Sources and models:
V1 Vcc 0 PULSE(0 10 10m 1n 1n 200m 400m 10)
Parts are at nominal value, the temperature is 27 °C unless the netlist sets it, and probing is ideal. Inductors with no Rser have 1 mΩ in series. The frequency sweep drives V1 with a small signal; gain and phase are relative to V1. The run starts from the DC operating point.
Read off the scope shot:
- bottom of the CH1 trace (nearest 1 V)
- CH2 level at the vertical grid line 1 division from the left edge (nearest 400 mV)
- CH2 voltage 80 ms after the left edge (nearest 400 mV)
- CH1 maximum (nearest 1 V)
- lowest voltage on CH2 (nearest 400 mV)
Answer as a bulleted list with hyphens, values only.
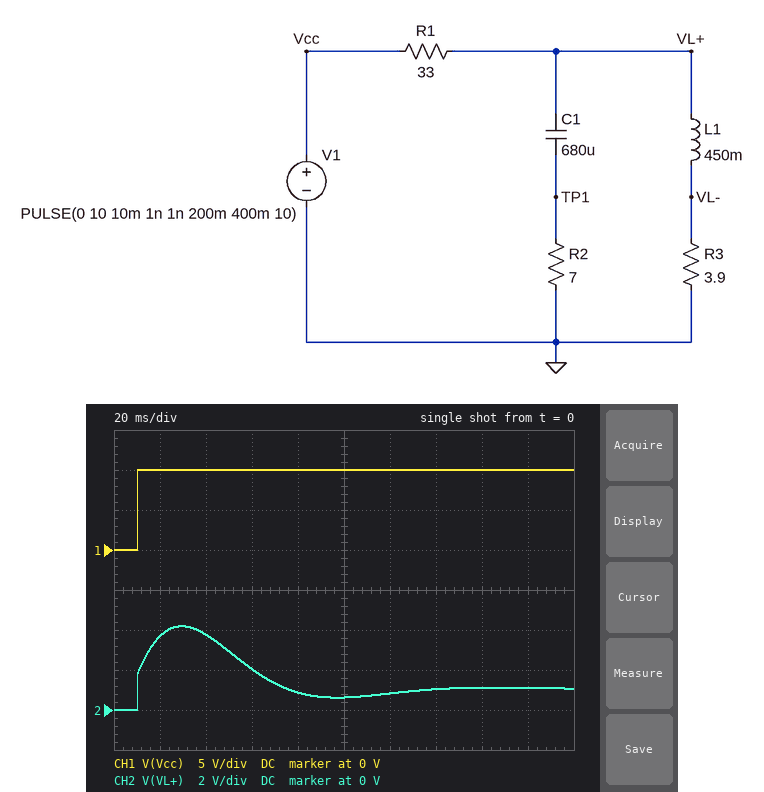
- 0 V
- 3.6 V
- 800 mV
- 10 V
- 0 V
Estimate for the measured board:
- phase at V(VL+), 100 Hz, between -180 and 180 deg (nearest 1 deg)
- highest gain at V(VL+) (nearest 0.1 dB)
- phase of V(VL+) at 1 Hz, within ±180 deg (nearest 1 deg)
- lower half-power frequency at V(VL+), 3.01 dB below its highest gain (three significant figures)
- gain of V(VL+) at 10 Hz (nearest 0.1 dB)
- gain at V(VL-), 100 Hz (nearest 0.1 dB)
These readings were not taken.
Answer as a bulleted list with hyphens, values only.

- -14 deg
- -3.6 dB
- 31 deg
- 5.26 Hz
- -3.8 dB
- -51.9 dB
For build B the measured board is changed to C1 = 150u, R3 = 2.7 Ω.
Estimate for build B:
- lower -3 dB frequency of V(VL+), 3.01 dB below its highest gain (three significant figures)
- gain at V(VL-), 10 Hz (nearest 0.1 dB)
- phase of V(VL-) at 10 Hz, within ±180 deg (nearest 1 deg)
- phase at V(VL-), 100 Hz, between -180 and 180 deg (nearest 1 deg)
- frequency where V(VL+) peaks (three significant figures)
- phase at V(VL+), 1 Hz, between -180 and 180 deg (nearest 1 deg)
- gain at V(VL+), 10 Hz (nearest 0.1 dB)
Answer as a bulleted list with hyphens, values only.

- 8.76 Hz
- -23.4 dB
- -48 deg
- -130 deg
- 18.4 Hz
- 42 deg
- -3.0 dB
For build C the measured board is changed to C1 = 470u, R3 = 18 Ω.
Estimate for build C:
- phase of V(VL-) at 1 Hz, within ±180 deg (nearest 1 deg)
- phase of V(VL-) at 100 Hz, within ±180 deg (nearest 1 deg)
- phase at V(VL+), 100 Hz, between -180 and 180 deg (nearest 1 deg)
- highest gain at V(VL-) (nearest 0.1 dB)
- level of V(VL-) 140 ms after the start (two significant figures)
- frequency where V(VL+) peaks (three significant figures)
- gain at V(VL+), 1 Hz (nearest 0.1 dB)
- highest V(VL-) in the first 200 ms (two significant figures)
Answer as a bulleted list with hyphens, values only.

- -5 deg
- -106 deg
- -20 deg
- -9.0 dB
- 3.5 V
- 11.3 Hz
- -8.9 dB
- 3.7 V
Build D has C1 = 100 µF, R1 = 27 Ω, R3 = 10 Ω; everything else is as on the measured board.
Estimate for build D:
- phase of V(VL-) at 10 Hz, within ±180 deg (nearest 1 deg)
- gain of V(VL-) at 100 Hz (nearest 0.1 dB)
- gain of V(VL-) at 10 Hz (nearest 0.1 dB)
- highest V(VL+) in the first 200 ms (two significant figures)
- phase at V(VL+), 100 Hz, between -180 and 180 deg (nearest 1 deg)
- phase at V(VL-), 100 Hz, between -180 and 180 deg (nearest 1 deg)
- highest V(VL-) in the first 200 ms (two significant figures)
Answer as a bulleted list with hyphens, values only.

- -43 deg
- -35.5 dB
- -12.9 dB
- 7.5 V
- -39 deg
- -127 deg
- 2.7 V
